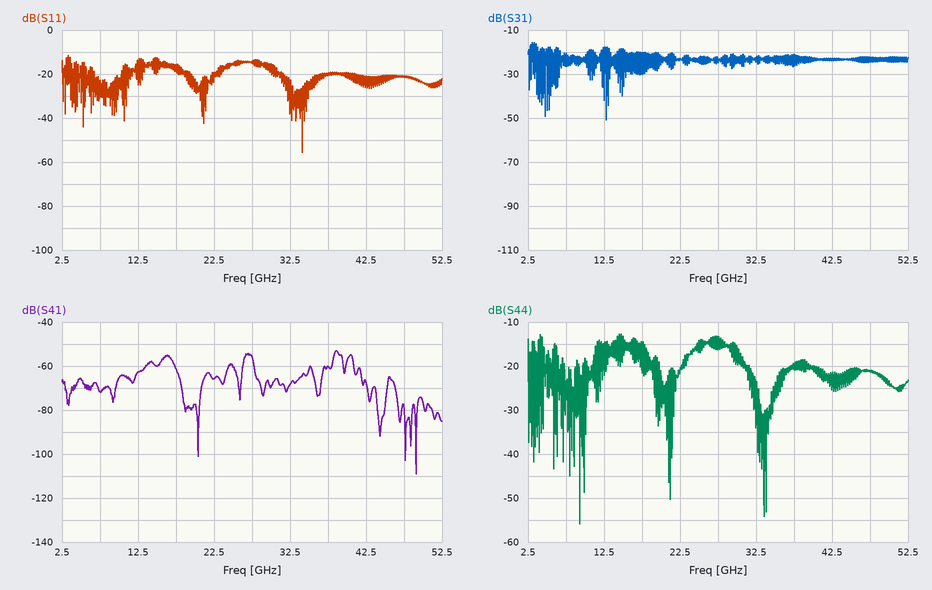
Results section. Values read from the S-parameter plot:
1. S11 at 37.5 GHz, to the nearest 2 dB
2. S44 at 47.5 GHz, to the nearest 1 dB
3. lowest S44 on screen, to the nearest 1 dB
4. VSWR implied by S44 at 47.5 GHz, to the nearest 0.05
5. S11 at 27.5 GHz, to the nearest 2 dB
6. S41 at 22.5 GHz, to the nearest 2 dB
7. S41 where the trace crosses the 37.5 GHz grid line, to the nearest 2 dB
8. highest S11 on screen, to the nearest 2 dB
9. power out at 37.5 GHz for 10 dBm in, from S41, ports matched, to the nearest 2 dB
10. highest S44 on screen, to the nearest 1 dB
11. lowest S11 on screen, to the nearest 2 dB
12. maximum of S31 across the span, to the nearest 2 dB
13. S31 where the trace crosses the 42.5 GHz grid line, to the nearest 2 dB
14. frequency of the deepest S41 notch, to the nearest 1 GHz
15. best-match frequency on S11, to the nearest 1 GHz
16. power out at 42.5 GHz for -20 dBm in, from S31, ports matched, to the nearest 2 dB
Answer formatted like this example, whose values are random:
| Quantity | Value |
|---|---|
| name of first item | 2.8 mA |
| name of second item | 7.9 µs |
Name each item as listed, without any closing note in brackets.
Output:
| Quantity | Value |
|---|---|
| S11 at 37.5 GHz, to the nearest 2 dB | -20 dB |
| S44 at 47.5 GHz, to the nearest 1 dB | -21 dB |
| lowest S44 on screen, to the nearest 1 dB | -56 dB |
| VSWR implied by S44 at 47.5 GHz, to the nearest 0.05 | 1.20 |
| S11 at 27.5 GHz, to the nearest 2 dB | -14 dB |
| S41 at 22.5 GHz, to the nearest 2 dB | -66 dB |
| S41 where the trace crosses the 37.5 GHz grid line, to the nearest 2 dB | -60 dB |
| highest S11 on screen, to the nearest 2 dB | -12 dB |
| power out at 37.5 GHz for 10 dBm in, from S41, ports matched, to the nearest 2 dB | -50 dBm |
| highest S44 on screen, to the nearest 1 dB | -13 dB |
| lowest S11 on screen, to the nearest 2 dB | -56 dB |
| maximum of S31 across the span, to the nearest 2 dB | -16 dB |
| S31 where the trace crosses the 42.5 GHz grid line, to the nearest 2 dB | -24 dB |
| frequency of the deepest S41 notch, to the nearest 1 GHz | 49 GHz |
| best-match frequency on S11, to the nearest 1 GHz | 34 GHz |
| power out at 42.5 GHz for -20 dBm in, from S31, ports matched, to the nearest 2 dB | -44 dBm |
